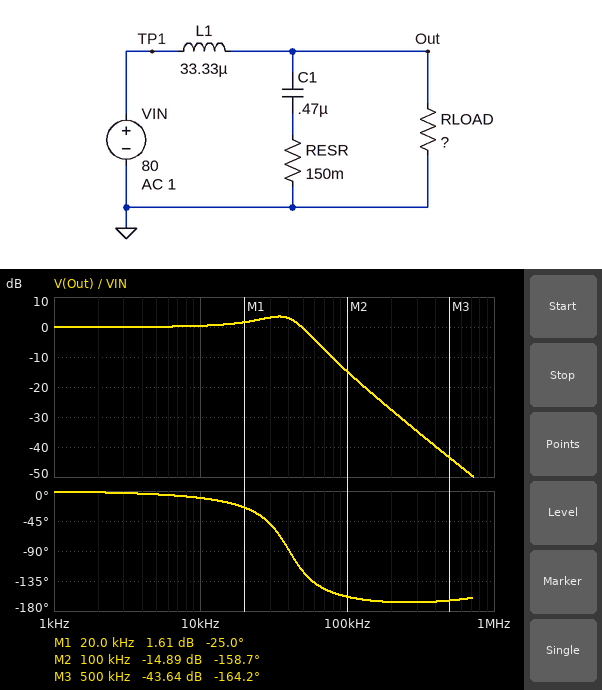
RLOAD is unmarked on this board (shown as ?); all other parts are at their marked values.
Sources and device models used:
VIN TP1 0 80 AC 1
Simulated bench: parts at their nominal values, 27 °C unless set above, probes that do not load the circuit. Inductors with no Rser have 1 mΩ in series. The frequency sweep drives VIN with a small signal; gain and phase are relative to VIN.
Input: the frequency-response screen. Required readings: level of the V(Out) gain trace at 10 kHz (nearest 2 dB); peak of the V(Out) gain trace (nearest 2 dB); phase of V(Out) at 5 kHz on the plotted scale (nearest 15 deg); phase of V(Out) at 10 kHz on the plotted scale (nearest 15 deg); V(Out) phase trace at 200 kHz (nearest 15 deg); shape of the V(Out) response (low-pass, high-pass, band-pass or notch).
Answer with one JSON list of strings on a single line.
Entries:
["0 dB", "4 dB", "0 deg", "-15 deg", "-165 deg", "low-pass"]
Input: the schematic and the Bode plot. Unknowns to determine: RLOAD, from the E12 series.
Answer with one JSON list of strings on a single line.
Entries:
["12 Ω"]
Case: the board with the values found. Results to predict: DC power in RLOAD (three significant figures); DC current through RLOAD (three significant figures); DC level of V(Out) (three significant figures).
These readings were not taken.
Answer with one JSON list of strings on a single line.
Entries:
["533 W", "6.67 A", "80.0 V"]
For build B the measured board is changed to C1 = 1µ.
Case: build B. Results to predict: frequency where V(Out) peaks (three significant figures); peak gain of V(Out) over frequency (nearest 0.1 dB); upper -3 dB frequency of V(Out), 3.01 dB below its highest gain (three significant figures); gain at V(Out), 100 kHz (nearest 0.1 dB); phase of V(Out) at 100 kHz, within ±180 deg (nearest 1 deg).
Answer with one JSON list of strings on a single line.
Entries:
["25.6 kHz", "6.2 dB", "32.0 kHz", "-21.9 dB", "-166 deg"]
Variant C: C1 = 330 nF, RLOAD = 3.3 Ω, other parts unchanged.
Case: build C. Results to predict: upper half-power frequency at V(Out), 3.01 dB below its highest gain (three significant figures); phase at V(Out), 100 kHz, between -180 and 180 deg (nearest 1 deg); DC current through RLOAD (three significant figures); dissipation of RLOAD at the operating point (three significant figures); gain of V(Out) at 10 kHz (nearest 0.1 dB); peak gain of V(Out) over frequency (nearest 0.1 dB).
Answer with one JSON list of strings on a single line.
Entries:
["17.6 kHz", "-117 deg", "24.2 A", "1.94 kW", "-1.2 dB", "0 dB"]
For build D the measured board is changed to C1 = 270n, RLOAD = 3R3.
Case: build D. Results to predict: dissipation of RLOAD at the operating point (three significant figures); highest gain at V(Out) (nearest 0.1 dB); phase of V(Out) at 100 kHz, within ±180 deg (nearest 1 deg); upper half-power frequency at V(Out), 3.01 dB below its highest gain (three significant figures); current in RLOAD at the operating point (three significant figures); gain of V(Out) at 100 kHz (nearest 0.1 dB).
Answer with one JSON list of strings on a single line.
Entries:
["1.94 kW", "0 dB", "-112 deg", "17.3 kHz", "24.2 A", "-16.8 dB"]
